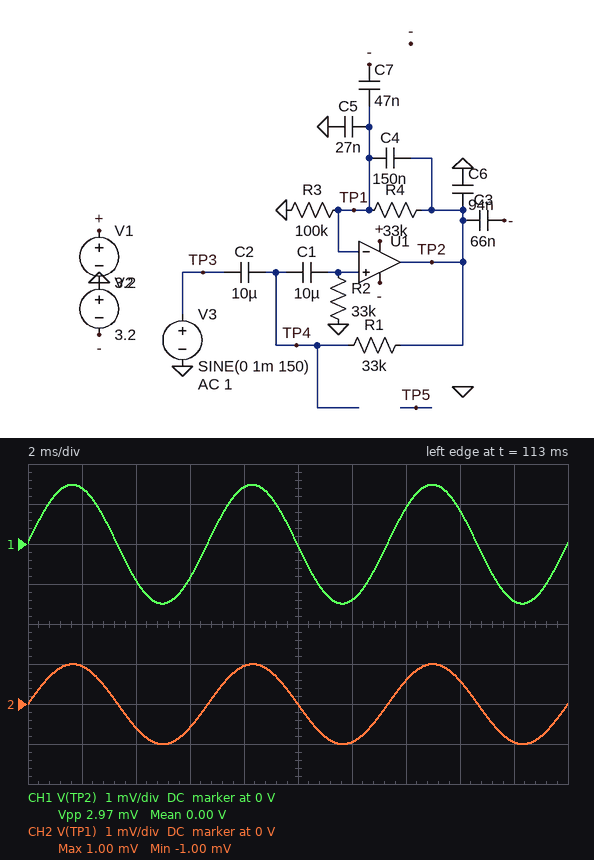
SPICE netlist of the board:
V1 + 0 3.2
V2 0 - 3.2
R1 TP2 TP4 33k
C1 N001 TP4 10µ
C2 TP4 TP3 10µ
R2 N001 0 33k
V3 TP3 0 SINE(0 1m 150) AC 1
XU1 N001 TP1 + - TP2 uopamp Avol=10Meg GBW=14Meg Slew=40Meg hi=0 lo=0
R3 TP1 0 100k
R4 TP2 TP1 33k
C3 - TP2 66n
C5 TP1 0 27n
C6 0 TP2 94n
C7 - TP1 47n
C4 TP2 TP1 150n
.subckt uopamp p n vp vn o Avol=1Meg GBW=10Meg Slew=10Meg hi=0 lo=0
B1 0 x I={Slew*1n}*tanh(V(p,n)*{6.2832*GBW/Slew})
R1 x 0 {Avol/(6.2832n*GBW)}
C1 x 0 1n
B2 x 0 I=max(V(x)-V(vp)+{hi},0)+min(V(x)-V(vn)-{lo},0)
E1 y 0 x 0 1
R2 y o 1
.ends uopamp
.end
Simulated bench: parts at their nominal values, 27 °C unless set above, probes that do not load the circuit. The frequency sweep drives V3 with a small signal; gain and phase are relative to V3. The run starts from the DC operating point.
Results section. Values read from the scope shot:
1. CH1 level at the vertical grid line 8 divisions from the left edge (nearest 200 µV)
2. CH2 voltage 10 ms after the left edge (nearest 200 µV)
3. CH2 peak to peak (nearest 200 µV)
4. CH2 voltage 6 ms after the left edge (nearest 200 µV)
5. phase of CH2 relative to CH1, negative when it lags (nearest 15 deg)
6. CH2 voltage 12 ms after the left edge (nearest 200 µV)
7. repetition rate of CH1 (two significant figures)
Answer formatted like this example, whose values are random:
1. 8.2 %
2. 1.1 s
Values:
1. 800 µV
2. 0 V
3. 2.0 mV
4. -600 µV
5. 0 deg
6. -1.0 mV
7. 150 Hz
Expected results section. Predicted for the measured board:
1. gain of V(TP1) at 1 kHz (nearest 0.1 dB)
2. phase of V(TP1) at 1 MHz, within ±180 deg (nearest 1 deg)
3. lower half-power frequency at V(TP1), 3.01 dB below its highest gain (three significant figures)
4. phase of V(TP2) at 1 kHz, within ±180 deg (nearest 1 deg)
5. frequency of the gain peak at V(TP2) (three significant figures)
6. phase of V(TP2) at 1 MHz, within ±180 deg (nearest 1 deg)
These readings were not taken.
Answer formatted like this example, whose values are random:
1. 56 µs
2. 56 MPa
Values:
1. 0 dB
2. -7 deg
3. 2.20 MHz
4. 0 deg
5. 2.61 MHz
6. -7 deg
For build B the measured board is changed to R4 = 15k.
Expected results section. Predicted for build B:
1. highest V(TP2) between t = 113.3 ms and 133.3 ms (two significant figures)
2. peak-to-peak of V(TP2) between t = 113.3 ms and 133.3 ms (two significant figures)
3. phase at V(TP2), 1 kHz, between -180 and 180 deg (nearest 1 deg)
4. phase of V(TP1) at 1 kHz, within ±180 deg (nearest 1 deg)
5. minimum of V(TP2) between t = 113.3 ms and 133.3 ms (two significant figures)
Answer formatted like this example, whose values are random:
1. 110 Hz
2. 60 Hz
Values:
1. 1.4 mV
2. 2.9 mV
3. 1 deg
4. 0 deg
5. -1.4 mV
